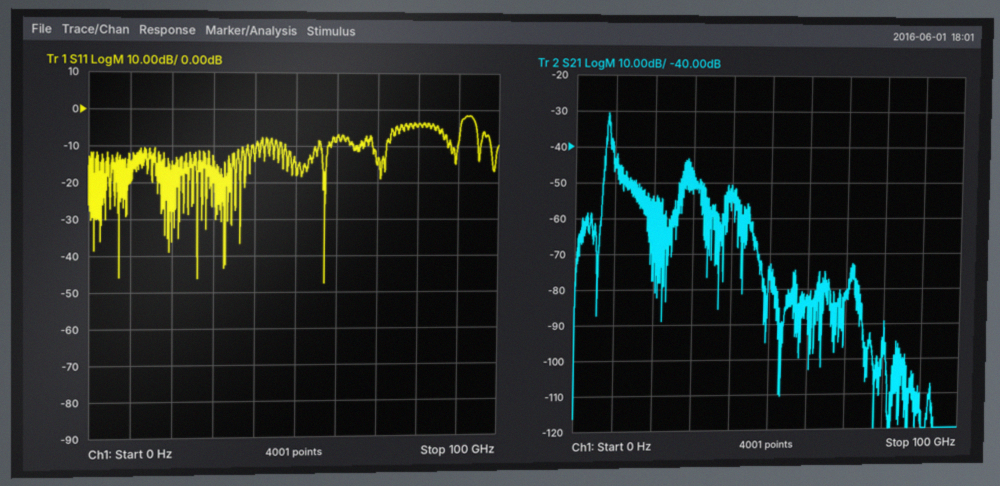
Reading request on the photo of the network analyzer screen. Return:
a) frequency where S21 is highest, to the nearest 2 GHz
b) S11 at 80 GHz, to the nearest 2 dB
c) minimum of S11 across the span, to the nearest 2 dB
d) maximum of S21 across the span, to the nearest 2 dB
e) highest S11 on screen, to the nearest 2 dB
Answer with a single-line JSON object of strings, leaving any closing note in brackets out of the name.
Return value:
{"frequency where S21 is highest, to the nearest 2 GHz": "8 GHz", "S11 at 80 GHz, to the nearest 2 dB": "-4 dB", "minimum of S11 across the span, to the nearest 2 dB": "-48 dB", "maximum of S21 across the span, to the nearest 2 dB": "-30 dB", "highest S11 on screen, to the nearest 2 dB": "-2 dB"}
